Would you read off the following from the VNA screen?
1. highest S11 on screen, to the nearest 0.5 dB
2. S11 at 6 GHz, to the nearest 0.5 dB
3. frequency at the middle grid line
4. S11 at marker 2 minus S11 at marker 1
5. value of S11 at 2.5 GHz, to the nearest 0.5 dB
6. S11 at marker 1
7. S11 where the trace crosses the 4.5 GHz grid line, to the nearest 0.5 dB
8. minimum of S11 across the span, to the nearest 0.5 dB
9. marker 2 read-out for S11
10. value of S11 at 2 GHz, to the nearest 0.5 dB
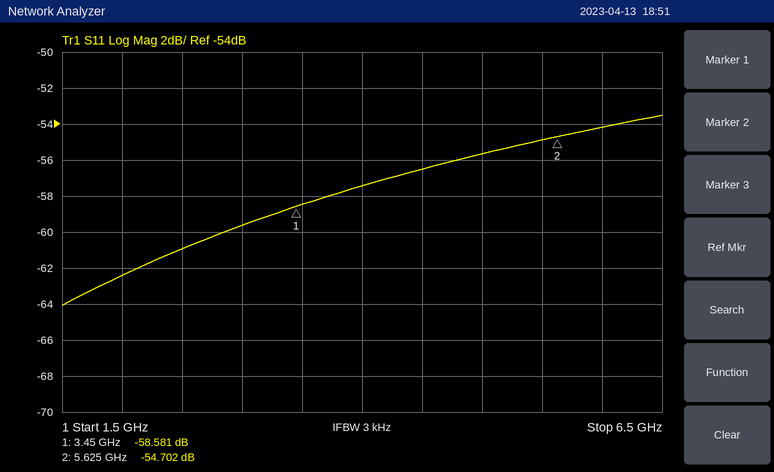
-53.5 dB
-54.0 dB
4 GHz
3.879 dB
-61.0 dB
-58.581 dB
-56.5 dB
-64.0 dB
-54.702 dB
-62.5 dB
